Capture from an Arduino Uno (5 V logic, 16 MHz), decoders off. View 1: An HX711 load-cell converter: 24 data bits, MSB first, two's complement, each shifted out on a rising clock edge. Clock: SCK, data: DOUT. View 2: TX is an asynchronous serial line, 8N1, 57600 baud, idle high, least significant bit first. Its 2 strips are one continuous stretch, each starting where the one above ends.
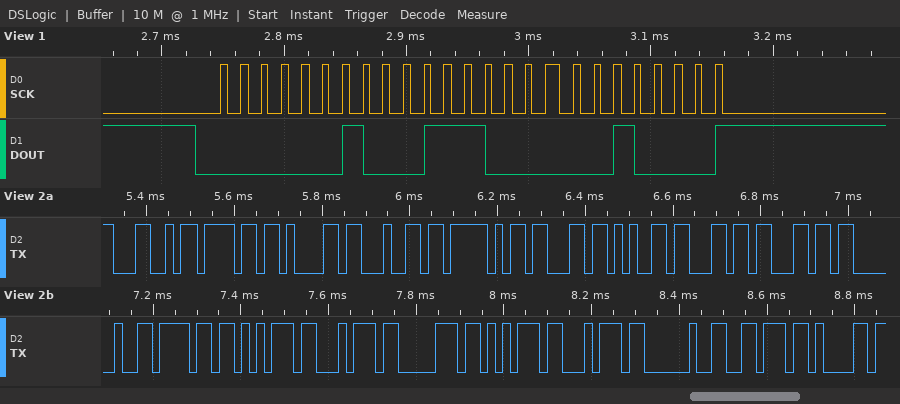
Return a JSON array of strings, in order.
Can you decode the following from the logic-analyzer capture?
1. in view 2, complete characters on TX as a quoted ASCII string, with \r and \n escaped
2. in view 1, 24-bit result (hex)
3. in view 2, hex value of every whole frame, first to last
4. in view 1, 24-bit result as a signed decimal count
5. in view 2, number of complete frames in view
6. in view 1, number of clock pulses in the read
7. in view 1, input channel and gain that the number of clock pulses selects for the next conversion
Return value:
["\"Load_cell output va\"", "0x023810", "4C 6F 61 64 5F 63 65 6C 6C 20 6F 75 74 70 75 74 20 76 61", "145424", "19", "25", "channel A, gain 128"]
